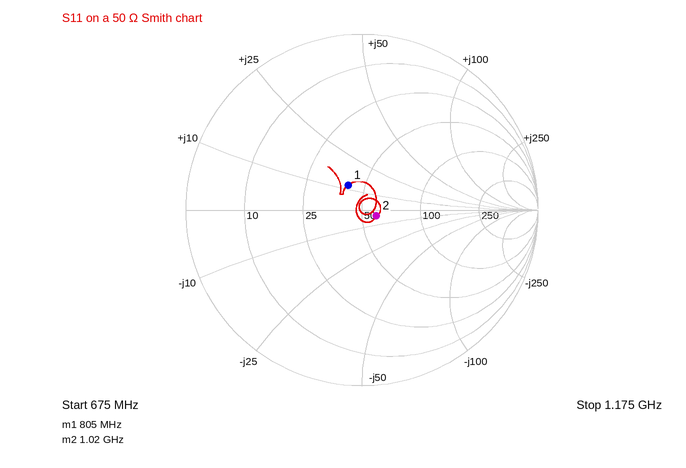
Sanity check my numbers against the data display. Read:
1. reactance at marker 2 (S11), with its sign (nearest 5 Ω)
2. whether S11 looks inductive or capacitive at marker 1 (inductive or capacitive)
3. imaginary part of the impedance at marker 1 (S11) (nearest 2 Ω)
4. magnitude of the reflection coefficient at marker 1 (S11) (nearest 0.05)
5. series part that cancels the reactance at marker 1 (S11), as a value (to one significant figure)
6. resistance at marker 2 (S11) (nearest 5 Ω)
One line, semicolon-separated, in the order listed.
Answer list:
-5 Ω; inductive; +12 Ω; 0.15; 20 pF; 60 Ω
